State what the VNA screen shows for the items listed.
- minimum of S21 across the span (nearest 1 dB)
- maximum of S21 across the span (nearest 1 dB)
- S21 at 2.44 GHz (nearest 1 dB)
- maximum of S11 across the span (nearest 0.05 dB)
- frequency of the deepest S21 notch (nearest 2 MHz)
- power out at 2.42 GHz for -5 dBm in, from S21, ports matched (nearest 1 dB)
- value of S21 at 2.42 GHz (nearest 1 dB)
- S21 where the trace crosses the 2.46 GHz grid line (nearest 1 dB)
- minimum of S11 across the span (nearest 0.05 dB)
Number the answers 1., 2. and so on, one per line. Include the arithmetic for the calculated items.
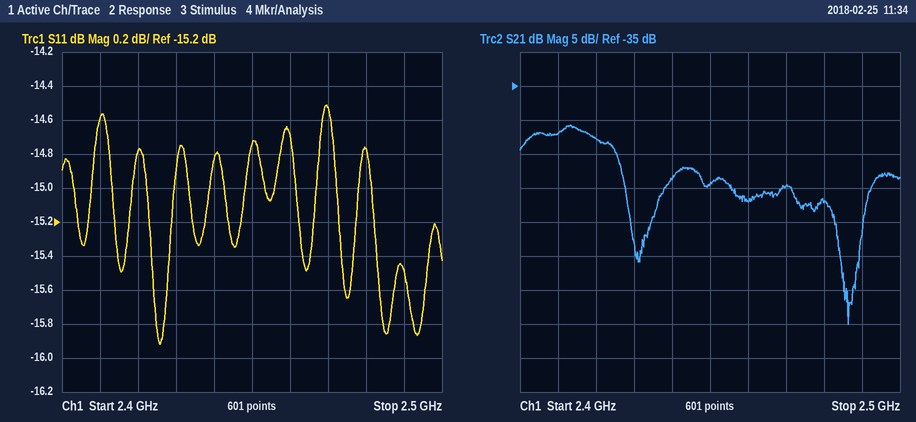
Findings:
1. -70 dB
2. -41 dB
3. -49 dB
4. -14.50 dB
5. 2.486 GHz
6. -5 dBm + (-43 dB) = -48 dBm
7. -43 dB
8. -52 dB
9. -15.90 dB
